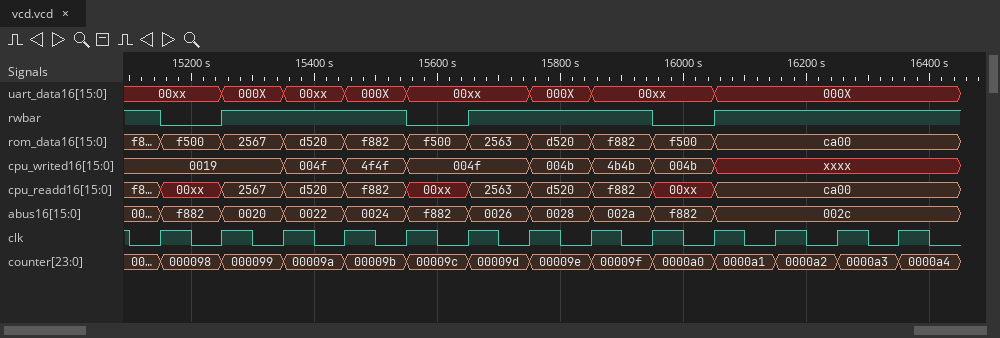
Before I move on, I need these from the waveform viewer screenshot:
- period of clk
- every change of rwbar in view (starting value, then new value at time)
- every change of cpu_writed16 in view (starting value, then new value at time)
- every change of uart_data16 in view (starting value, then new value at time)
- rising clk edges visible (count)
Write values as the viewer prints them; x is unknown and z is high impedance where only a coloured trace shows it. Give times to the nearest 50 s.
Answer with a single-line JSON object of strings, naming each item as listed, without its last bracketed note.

{"period of clk": "100 s", "every change of rwbar in view": "1, 0 at 15150 s, 1 at 15250 s, 0 at 15550 s, 1 at 15650 s, 0 at 15950 s, 1 at 16050 s", "every change of cpu_writed16 in view": "0019, 004f at 15350 s, 4f4f at 15450 s, 004f at 15550 s, 004b at 15750 s, 4b4b at 15850 s, 004b at 15950 s, xxxx at 16050 s", "every change of uart_data16 in view": "00xx, 000X at 15250 s, 00xx at 15350 s, 000X at 15450 s, 00xx at 15550 s, 000X at 15750 s, 00xx at 15850 s, 000X at 16050 s", "rising clk edges visible": "13"}
